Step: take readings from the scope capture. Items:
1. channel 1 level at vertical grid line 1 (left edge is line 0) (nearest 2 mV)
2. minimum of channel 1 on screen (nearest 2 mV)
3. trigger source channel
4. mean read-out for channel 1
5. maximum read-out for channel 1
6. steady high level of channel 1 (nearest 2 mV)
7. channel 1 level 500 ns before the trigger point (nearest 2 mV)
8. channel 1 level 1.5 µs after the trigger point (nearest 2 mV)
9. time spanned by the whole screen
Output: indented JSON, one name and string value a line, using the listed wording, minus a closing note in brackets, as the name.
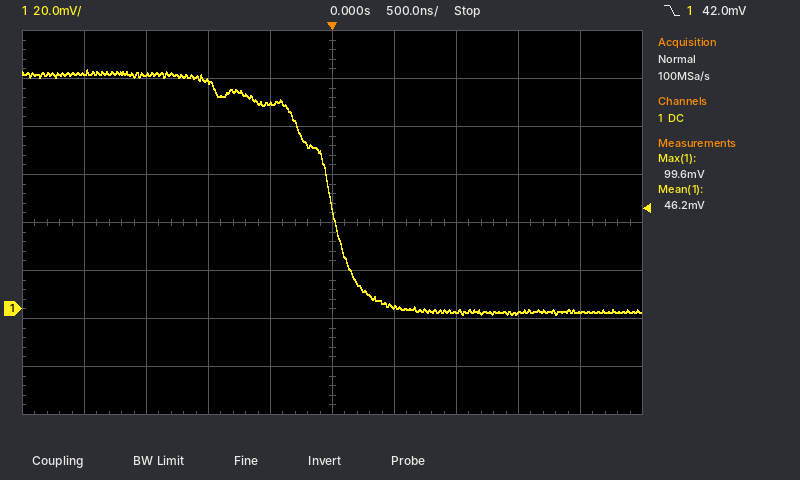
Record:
{
  "channel 1 level at vertical grid line 1 (left edge is line 0)": "98 mV",
  "minimum of channel 1 on screen": "-2 mV",
  "trigger source channel": "channel 1",
  "mean read-out for channel 1": "46.2 mV",
  "maximum read-out for channel 1": "99.6 mV",
  "steady high level of channel 1": "98 mV",
  "channel 1 level 500 ns before the trigger point": "86 mV",
  "channel 1 level 1.5 µs after the trigger point": "-2 mV",
  "time spanned by the whole screen": "5 µs"
}
